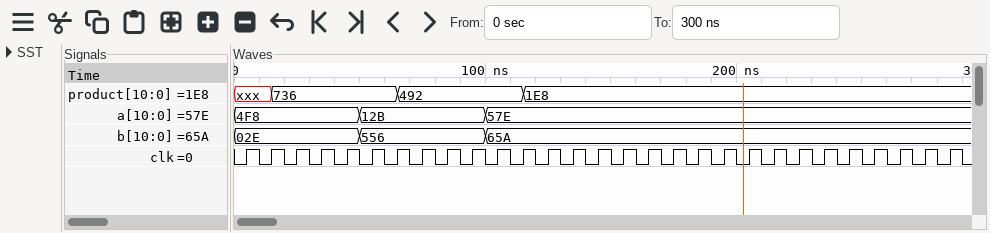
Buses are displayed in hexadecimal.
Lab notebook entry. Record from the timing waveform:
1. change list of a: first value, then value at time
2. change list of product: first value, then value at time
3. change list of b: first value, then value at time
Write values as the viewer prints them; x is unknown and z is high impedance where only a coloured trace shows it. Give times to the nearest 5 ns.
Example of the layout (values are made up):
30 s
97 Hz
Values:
4F8, 12B at 50 ns, 57E at 100 ns
xxx, 736 at 15 ns, 492 at 65 ns, 1E8 at 115 ns
02E, 556 at 50 ns, 65A at 100 ns
